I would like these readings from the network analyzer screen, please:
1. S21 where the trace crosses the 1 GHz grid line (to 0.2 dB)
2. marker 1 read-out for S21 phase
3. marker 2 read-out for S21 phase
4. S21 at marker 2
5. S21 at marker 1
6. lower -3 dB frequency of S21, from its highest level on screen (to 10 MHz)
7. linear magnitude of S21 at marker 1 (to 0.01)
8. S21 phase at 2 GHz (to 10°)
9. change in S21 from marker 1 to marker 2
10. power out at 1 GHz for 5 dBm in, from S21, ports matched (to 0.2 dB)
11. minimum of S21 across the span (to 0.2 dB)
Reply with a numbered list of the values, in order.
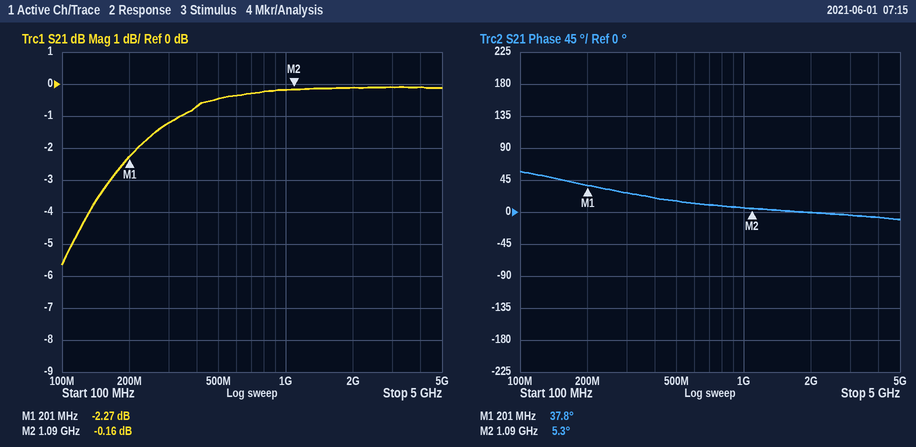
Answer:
1. -0.2 dB
2. 37.8°
3. 5.3°
4. -0.16 dB
5. -2.27 dB
6. 160 MHz
7. 0.77
8. 0°
9. 2.11 dB
10. 4.8 dBm
11. -5.6 dB
